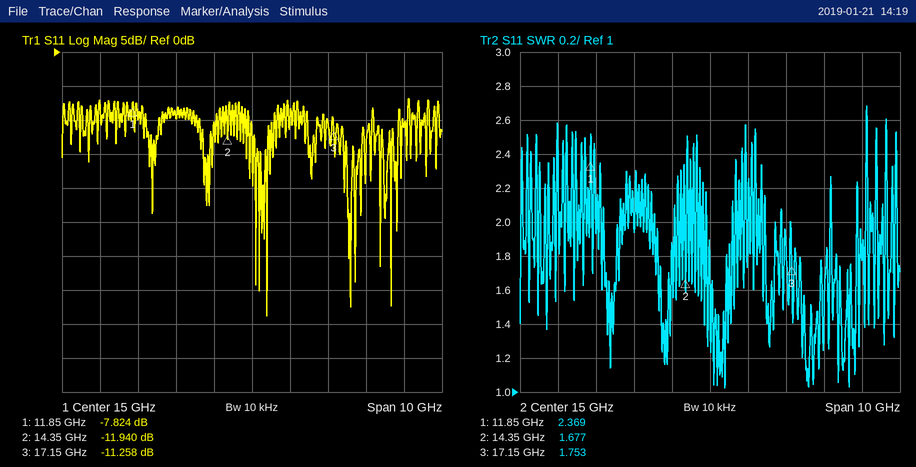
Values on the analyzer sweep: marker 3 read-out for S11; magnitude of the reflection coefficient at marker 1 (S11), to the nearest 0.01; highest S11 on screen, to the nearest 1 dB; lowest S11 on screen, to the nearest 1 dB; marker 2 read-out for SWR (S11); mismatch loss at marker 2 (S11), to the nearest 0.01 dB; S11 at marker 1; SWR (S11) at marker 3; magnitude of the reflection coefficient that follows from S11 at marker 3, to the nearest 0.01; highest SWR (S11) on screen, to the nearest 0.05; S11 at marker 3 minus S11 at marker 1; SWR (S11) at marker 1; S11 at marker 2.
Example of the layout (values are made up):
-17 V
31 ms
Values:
-11.258 dB
0.41
-7 dB
-39 dB
1.677
0.29 dB
-7.824 dB
1.753
0.27
2.70
-3.434 dB
2.369
-11.940 dB
